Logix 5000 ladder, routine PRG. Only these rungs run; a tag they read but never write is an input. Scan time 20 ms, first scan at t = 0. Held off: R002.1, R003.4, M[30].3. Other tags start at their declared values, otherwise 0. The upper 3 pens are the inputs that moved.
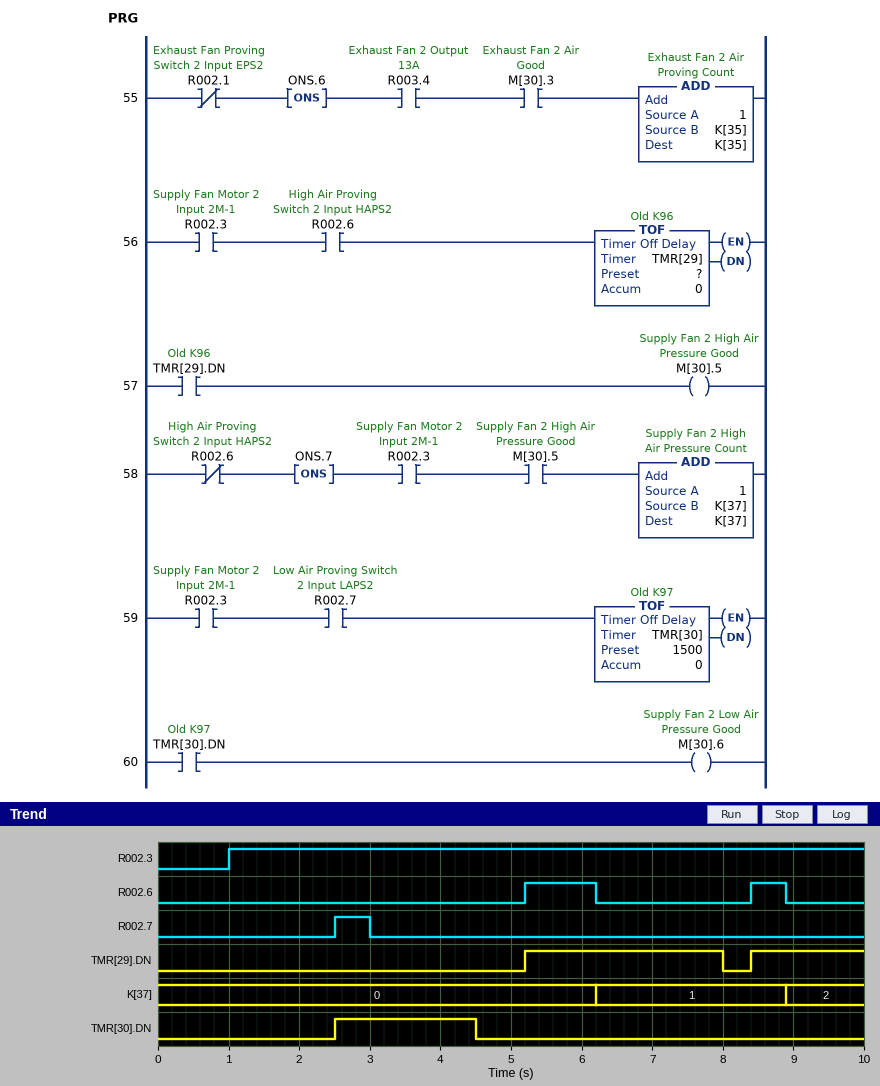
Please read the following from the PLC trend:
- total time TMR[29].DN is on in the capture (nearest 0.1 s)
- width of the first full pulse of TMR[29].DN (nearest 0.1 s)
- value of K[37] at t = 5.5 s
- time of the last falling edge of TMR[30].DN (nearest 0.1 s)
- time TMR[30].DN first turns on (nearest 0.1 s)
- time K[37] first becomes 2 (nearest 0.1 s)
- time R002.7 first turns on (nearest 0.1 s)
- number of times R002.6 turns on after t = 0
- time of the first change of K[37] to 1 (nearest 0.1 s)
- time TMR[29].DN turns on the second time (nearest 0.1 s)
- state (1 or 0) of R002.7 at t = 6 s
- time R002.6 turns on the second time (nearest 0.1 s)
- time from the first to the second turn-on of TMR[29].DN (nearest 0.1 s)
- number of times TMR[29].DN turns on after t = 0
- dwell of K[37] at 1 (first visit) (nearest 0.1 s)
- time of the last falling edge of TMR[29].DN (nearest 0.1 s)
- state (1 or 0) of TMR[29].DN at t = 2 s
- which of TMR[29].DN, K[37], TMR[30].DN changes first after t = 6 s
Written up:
4.4 s
2.8 s
0
4.5 s
2.5 s
8.9 s
2.5 s
2
6.2 s
8.4 s
0
8.4 s
3.2 s
2
2.7 s
8.0 s
0
K[37]
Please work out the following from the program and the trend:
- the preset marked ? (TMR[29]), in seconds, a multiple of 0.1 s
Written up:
1.8 s
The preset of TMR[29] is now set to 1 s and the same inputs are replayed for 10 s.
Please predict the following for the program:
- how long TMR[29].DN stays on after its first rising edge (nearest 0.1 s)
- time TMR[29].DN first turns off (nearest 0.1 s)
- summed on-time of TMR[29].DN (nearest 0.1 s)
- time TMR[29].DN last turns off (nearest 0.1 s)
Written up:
2.0 s
7.2 s
3.5 s
9.9 s
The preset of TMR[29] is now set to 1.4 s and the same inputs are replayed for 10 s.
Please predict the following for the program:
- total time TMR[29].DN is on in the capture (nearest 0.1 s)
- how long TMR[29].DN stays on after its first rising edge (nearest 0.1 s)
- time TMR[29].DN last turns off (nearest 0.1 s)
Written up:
4.0 s
2.4 s
7.6 s
